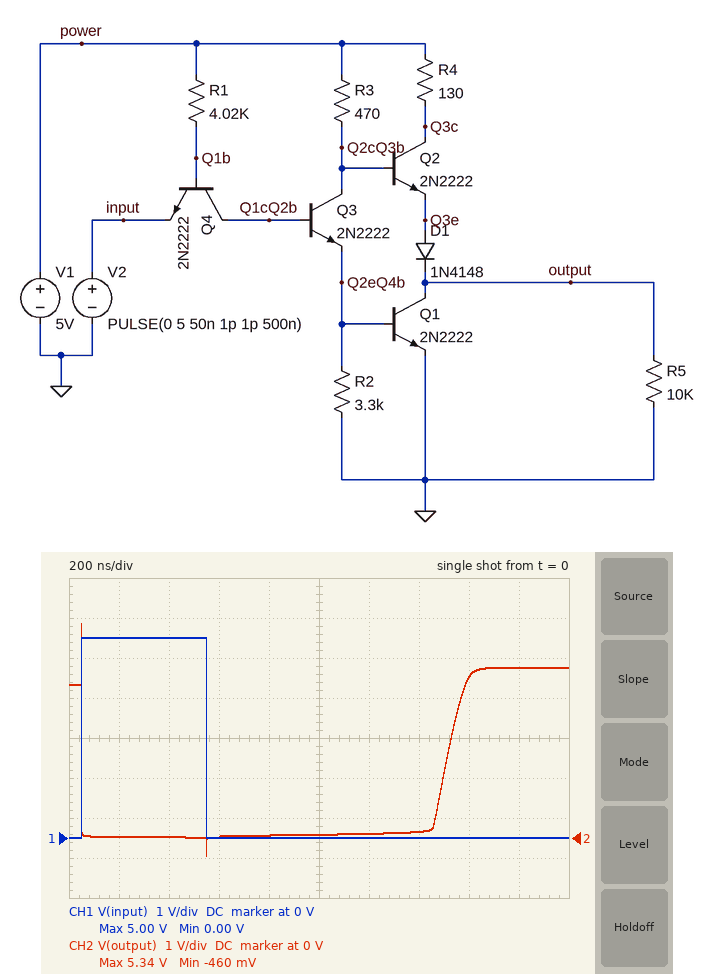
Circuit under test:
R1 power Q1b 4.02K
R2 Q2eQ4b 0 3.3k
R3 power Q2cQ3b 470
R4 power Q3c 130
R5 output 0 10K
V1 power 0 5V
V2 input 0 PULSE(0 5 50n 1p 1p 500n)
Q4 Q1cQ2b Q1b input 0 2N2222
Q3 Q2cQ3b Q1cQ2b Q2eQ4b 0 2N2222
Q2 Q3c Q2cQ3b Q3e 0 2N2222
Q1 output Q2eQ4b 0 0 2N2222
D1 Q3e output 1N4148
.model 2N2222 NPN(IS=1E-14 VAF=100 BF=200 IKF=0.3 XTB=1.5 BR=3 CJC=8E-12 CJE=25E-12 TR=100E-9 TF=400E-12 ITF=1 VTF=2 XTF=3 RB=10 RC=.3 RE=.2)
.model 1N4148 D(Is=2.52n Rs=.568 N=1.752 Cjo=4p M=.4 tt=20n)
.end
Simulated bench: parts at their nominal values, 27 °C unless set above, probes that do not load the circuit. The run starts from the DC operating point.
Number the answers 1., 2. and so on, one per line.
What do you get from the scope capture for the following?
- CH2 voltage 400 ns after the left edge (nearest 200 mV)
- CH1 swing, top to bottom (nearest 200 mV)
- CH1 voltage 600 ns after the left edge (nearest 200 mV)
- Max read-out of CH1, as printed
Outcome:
1. 0 V
2. 5.0 V
3. 0 V
4. 5.00 V
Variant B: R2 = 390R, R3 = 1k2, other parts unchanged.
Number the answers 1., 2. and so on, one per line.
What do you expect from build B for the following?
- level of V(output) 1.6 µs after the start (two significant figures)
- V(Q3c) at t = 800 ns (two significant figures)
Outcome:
1. 3.8 V
2. 990 mV
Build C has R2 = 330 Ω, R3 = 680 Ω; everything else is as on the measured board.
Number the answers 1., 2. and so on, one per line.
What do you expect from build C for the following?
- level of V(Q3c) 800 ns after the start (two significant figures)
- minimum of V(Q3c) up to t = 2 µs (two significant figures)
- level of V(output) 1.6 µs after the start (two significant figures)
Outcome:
1. 930 mV
2. 920 mV
3. 3.8 V
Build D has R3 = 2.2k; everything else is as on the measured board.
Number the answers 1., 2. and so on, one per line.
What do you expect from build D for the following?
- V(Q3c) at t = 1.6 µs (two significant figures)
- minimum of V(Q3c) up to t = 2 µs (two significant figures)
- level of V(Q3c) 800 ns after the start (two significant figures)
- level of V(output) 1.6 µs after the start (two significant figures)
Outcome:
1. 4.9 V
2. 950 mV
3. 960 mV
4. 4.3 V
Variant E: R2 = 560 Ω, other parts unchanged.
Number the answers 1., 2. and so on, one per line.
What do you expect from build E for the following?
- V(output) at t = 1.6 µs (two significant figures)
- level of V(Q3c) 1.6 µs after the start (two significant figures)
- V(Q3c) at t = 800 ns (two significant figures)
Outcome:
1. 4.3 V
2. 4.8 V
3. 900 mV
